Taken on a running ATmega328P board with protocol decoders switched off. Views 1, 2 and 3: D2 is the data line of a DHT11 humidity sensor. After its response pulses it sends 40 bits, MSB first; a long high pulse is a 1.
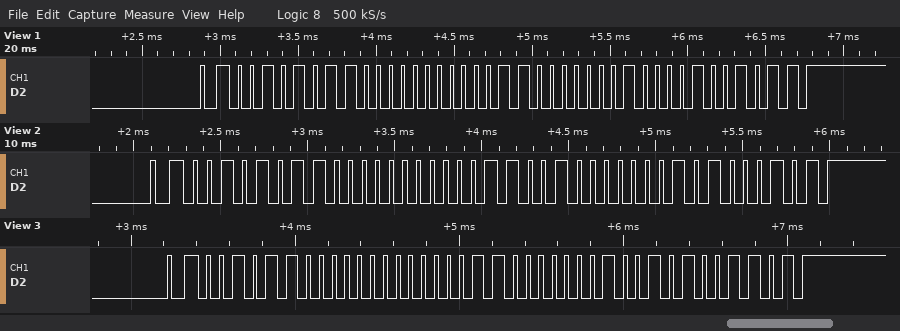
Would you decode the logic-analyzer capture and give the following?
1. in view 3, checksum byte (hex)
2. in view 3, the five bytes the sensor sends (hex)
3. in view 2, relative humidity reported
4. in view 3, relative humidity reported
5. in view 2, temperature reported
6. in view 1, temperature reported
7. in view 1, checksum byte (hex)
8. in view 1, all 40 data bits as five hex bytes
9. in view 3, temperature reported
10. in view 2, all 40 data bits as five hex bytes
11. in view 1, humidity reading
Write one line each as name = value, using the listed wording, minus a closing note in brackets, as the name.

in view 3, checksum byte = 0x4D
in view 3, the five bytes the sensor sends = 2C 00 18 09 4D
in view 2, relative humidity reported = 43 %
in view 3, relative humidity reported = 44 %
in view 2, temperature reported = 25.1 °C
in view 1, temperature reported = 24.8 °C
in view 1, checksum byte = 0x4B
in view 1, all 40 data bits as five hex bytes = 2B 00 18 08 4B
in view 3, temperature reported = 24.9 °C
in view 2, all 40 data bits as five hex bytes = 2B 00 19 01 45
in view 1, humidity reading = 43 %
